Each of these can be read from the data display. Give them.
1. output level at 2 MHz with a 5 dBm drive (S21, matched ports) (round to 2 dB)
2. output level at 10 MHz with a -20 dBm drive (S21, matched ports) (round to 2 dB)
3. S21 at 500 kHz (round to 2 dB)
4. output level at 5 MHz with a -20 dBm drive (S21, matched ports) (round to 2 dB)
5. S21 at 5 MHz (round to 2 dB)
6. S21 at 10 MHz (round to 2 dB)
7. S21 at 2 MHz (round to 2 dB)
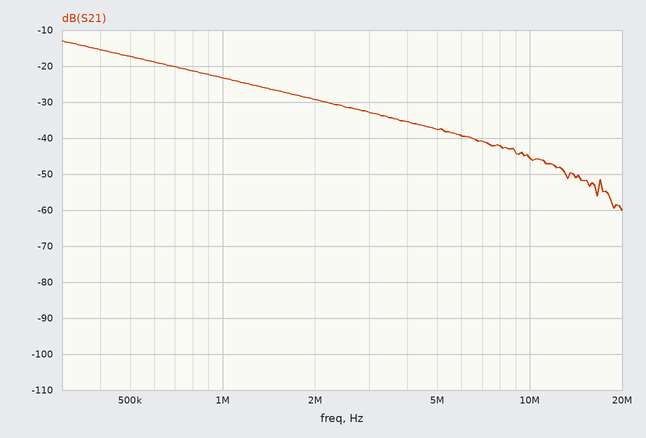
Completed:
-24 dBm
-66 dBm
-18 dB
-58 dBm
-38 dB
-46 dB
-30 dB
